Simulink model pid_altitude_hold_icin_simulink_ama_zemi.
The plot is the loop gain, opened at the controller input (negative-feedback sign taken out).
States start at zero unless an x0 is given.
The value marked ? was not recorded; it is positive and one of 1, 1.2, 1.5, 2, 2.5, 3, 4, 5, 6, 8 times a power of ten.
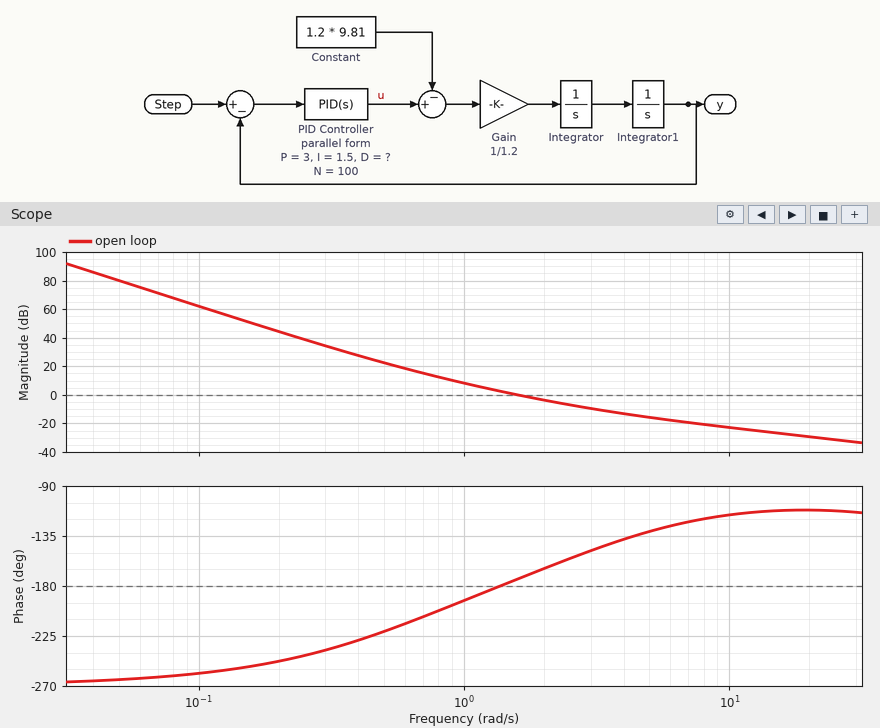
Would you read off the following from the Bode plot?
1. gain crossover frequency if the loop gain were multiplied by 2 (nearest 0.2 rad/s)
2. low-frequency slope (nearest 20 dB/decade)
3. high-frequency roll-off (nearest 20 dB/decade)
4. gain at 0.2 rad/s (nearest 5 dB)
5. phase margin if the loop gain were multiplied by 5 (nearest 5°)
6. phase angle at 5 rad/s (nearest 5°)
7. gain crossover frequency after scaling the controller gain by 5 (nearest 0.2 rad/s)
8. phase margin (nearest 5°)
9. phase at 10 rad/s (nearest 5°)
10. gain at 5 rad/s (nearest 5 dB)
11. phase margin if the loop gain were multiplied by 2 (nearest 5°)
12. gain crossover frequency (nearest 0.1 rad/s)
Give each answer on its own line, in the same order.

2.4 rad/s
-60 dB/decade
-20 dB/decade
45 dB
45°
-130°
4.2 rad/s
5°
-115°
-15 dB
20°
1.6 rad/s
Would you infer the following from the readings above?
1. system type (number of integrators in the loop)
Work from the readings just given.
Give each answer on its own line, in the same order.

3
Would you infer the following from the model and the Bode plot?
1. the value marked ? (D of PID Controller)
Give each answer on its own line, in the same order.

0.8
